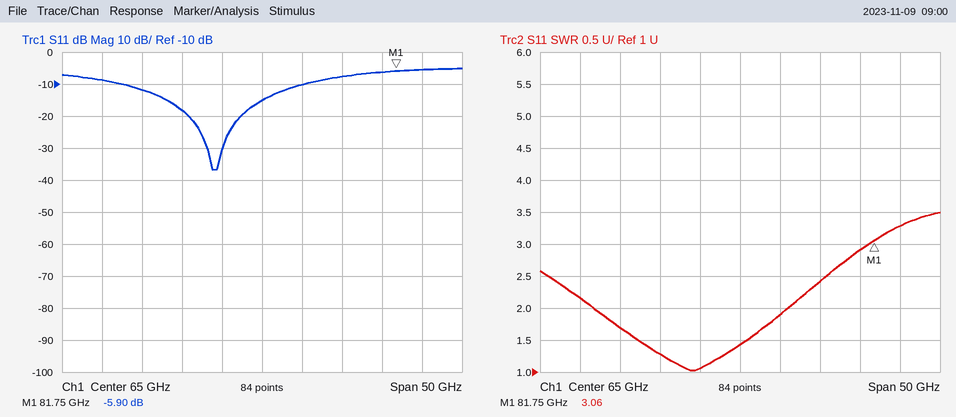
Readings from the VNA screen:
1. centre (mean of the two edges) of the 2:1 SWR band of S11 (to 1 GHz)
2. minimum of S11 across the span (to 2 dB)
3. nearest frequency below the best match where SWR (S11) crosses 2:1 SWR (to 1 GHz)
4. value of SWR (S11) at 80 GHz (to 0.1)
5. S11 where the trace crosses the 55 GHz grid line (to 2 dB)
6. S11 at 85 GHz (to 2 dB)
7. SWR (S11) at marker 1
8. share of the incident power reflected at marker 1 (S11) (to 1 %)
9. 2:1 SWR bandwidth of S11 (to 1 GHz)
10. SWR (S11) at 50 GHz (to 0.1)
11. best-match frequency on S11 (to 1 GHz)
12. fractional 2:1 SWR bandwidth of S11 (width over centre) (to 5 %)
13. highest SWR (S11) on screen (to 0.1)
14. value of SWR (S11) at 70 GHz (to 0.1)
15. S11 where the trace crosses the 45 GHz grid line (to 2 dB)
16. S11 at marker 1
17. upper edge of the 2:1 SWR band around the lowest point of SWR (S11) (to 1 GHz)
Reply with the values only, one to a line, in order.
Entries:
59 GHz
-36 dB
47 GHz
2.9
-18 dB
-6 dB
3.06
26 %
24 GHz
1.7
59 GHz
40 %
3.5
1.9
-8 dB
-5.90 dB
71 GHz
